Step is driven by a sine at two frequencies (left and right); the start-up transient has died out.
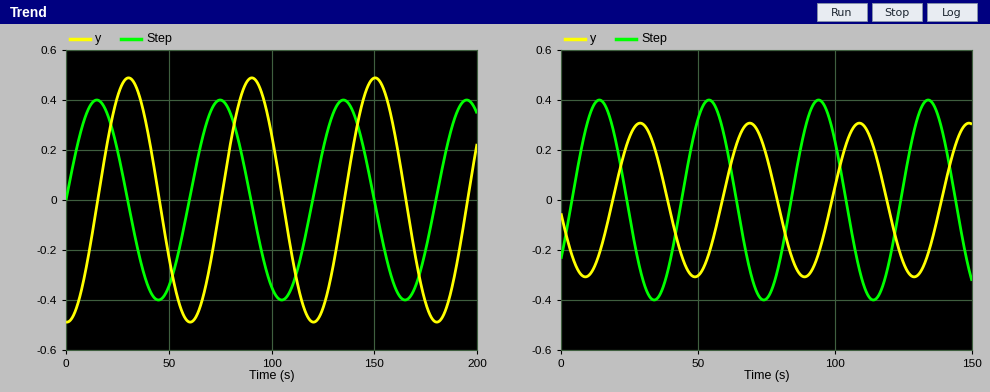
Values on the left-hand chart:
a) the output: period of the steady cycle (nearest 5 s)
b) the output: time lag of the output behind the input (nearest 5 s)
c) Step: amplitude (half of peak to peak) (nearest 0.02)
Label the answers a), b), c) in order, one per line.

a) 60 s
b) 15 s
c) 0.40
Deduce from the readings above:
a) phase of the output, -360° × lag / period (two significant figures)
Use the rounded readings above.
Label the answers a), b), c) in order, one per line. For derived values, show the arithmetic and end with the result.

a) -360 × 15 / 60 = -90°
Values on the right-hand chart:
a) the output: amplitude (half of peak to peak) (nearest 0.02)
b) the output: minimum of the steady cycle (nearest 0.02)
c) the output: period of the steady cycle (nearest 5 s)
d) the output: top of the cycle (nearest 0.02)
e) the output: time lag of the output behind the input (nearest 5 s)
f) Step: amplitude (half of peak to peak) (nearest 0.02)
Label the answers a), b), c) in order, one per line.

a) 0.30
b) -0.30
c) 40 s
d) 0.30
e) 15 s
f) 0.40
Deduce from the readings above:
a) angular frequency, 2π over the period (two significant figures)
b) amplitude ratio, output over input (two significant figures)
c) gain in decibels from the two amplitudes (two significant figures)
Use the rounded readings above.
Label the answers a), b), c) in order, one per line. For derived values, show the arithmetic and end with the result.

a) 2π / 40 = 0.16 rad/s
b) 0.3 / 0.4 = 0.75
c) 20 log10(0.3 / 0.4) = -2.5 dB
